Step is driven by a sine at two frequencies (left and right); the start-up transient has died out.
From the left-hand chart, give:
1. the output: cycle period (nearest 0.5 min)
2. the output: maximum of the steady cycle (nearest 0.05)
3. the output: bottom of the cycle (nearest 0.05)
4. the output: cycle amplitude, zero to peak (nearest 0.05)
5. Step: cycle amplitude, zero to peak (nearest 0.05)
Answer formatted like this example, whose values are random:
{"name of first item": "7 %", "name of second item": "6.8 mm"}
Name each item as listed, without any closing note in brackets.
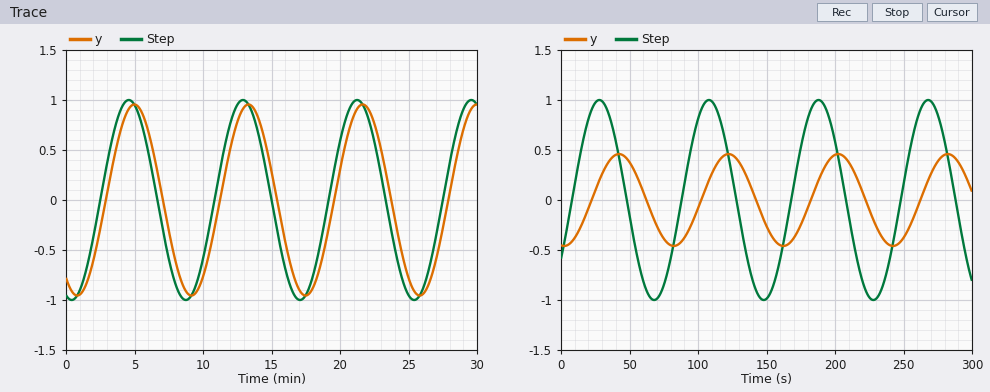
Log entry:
{"the output: cycle period": "8.5 min", "the output: maximum of the steady cycle": "0.95", "the output: bottom of the cycle": "-0.95", "the output: cycle amplitude, zero to peak": "0.95", "Step: cycle amplitude, zero to peak": "1.00"}
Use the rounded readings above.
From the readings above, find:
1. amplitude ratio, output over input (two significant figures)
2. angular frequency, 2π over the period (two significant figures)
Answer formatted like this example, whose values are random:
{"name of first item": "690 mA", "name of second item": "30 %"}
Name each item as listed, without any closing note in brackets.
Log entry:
{"amplitude ratio, output over input": "0.95", "angular frequency, 2π over the period": "0.74 rad/min"}
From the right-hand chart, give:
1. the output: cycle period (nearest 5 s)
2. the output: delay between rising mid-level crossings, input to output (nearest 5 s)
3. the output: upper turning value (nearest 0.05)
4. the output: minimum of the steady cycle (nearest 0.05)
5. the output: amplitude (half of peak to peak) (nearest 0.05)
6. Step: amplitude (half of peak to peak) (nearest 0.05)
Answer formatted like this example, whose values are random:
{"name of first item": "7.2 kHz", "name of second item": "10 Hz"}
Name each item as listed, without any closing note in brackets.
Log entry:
{"the output: cycle period": "80 s", "the output: delay between rising mid-level crossings, input to output": "15 s", "the output: upper turning value": "0.45", "the output: minimum of the steady cycle": "-0.45", "the output: amplitude (half of peak to peak)": "0.45", "Step: amplitude (half of peak to peak)": "1.00"}
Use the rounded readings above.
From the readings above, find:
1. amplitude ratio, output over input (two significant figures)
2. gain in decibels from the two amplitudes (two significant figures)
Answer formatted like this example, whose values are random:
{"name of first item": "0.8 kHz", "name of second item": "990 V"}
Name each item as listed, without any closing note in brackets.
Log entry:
{"amplitude ratio, output over input": "0.45", "gain in decibels from the two amplitudes": "-6.9 dB"}
